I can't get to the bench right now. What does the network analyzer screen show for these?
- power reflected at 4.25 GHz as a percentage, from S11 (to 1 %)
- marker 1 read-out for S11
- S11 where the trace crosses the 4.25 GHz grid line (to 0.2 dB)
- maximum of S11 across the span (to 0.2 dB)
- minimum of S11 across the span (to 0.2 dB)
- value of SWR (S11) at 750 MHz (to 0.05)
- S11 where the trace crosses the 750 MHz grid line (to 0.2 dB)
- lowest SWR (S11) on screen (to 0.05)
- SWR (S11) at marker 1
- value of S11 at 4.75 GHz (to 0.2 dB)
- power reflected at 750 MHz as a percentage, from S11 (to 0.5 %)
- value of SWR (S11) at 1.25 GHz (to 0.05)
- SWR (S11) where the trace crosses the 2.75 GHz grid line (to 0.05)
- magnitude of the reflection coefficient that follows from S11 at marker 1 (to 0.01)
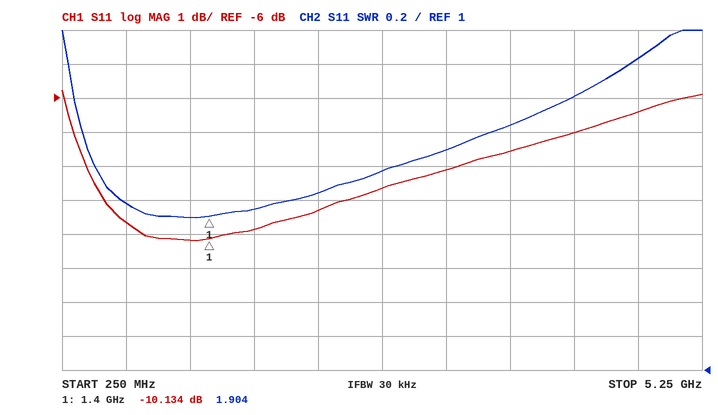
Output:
20 %
-10.134 dB
-7.0 dB
-5.8 dB
-10.2 dB
2.00
-9.6 dB
1.90
1.904
-6.4 dB
11.0 %
1.90
2.15
0.31
